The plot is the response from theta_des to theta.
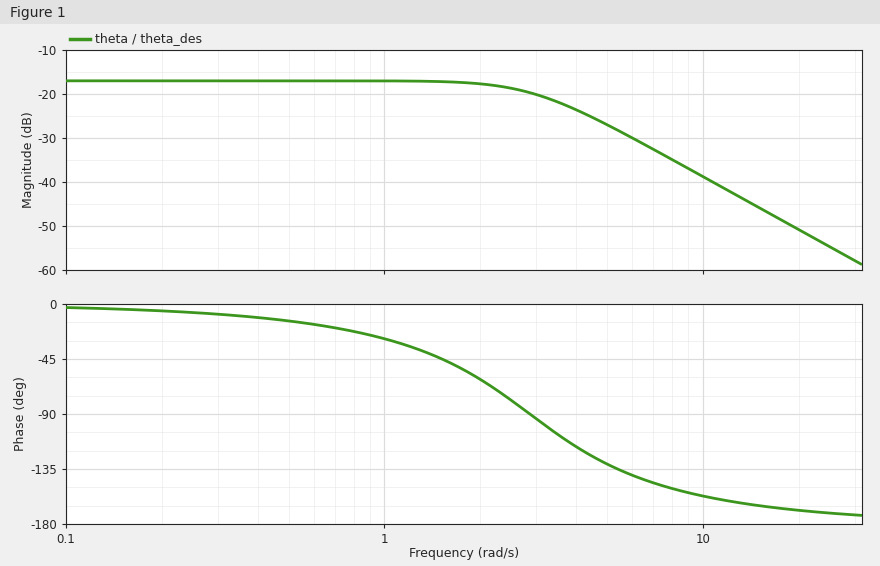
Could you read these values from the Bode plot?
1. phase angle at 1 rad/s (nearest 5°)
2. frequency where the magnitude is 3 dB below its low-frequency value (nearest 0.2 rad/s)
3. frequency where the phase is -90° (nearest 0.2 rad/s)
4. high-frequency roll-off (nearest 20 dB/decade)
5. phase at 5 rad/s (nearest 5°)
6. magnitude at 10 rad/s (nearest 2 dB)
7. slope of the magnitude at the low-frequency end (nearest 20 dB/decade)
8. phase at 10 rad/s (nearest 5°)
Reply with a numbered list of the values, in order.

1. -30°
2. 3.0 rad/s
3. 2.8 rad/s
4. -40 dB/decade
5. -130°
6. -38 dB
7. 0 dB/decade
8. -155°
